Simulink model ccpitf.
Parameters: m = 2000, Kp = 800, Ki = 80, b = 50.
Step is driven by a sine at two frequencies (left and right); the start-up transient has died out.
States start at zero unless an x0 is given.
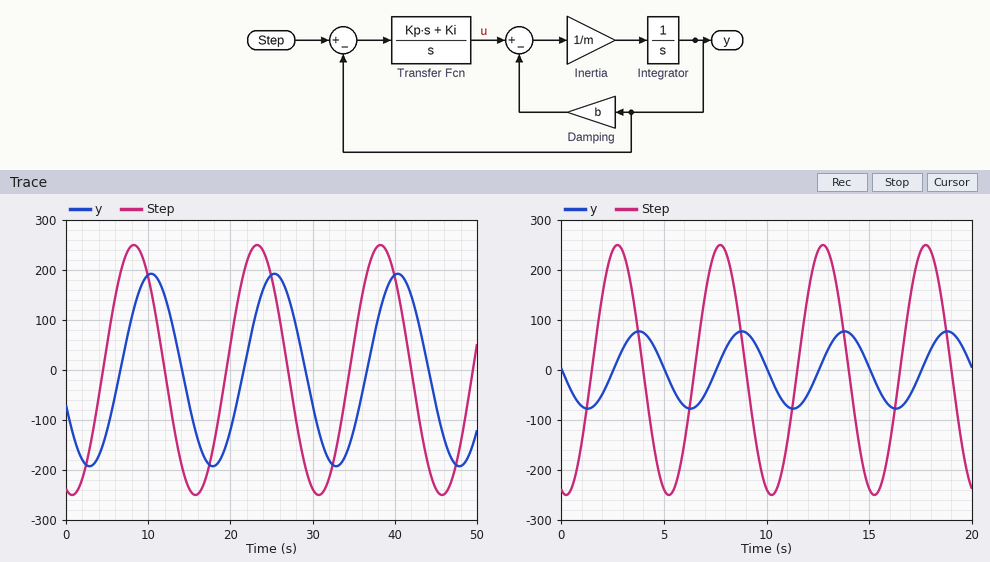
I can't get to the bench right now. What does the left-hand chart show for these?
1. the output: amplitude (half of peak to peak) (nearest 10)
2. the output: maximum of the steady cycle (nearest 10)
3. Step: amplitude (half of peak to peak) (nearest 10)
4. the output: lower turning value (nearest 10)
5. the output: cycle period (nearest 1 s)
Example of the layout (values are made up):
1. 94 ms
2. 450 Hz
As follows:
1. 190
2. 190
3. 250
4. -190
5. 15 s
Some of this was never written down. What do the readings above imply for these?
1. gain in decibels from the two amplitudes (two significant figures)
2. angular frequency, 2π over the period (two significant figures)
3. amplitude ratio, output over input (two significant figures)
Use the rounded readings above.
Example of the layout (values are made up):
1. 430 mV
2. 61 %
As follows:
1. -2.4 dB
2. 0.42 rad/s
3. 0.76
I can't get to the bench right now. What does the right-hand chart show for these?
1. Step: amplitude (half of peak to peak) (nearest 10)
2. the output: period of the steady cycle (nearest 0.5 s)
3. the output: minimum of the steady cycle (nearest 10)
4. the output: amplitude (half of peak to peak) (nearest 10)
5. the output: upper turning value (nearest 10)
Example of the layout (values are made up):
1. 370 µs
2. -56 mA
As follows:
1. 250
2. 5.0 s
3. -80
4. 80
5. 80
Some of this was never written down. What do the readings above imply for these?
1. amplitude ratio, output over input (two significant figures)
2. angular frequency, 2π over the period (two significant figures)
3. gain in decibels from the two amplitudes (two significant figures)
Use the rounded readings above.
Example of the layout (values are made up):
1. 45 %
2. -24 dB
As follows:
1. 0.32
2. 1.3 rad/s
3. -9.9 dB
